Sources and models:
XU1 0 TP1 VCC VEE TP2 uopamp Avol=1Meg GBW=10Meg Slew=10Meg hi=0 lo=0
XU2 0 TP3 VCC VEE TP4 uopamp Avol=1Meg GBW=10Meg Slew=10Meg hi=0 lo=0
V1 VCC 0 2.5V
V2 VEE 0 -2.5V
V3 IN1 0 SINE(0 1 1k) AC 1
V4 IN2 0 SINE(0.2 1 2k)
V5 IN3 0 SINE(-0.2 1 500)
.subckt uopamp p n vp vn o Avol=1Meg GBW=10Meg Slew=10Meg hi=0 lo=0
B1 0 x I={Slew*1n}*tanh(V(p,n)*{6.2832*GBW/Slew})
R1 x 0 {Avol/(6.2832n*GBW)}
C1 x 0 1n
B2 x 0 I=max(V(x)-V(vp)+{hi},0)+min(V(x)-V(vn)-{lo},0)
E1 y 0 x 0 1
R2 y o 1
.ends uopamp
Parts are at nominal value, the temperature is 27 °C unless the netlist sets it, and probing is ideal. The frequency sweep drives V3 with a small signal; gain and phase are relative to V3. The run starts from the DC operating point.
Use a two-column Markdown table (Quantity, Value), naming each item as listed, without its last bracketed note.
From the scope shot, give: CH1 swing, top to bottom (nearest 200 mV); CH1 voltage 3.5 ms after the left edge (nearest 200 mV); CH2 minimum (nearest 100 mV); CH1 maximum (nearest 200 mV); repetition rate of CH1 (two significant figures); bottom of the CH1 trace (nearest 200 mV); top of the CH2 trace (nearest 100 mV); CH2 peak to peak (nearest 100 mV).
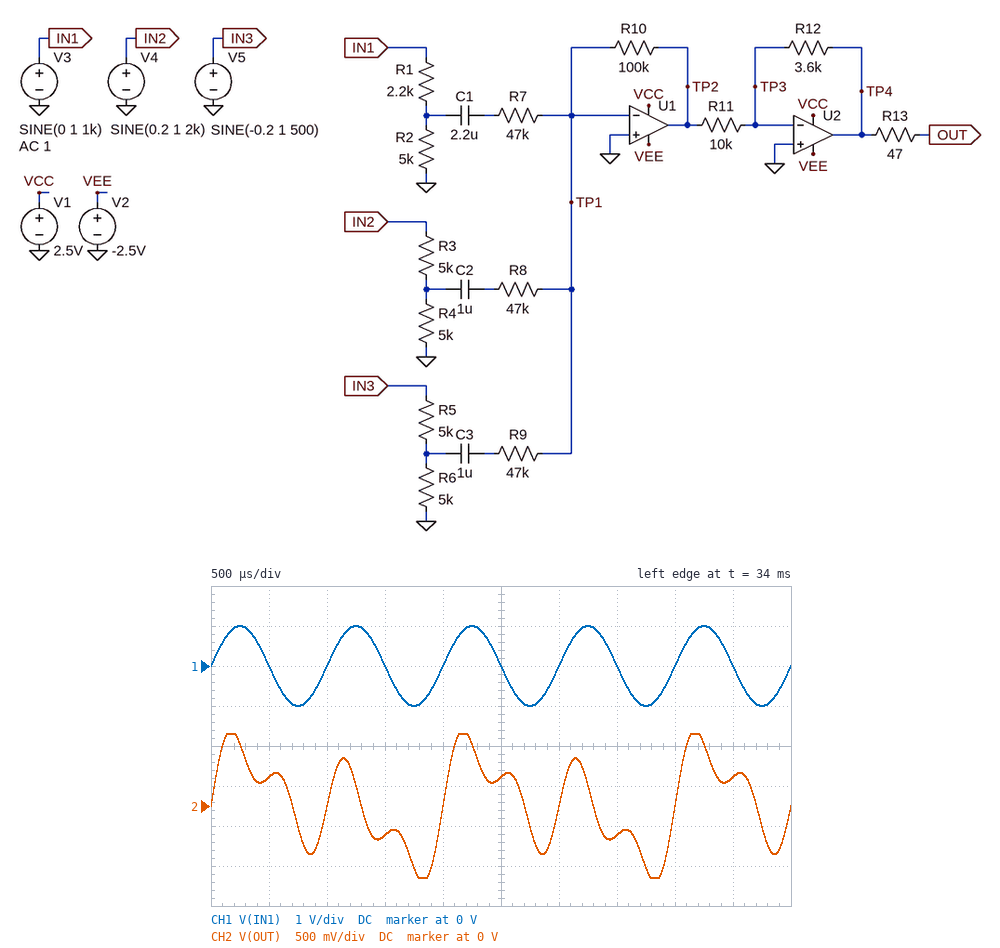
| Quantity | Value |
|---|---|
| CH1 swing, top to bottom | 2.0 V |
| CH1 voltage 3.5 ms after the left edge | 0 V |
| CH2 minimum | -900 mV |
| CH1 maximum | 1.0 V |
| repetition rate of CH1 | 1.0 kHz |
| bottom of the CH1 trace | -1.0 V |
| top of the CH2 trace | 900 mV |
| CH2 peak to peak | 1.8 V |
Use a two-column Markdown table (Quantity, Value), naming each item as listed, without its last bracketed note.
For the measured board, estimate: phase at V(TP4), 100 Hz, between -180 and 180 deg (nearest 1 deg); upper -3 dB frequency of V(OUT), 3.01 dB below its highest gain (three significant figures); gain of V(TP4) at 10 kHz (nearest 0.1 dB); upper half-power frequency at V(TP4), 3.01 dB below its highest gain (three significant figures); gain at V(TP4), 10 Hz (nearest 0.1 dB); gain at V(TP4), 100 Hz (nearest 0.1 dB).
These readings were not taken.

| Quantity | Value |
|---|---|
| phase at V(TP4), 100 Hz, between -180 and 180 deg | 1 deg |
| upper -3 dB frequency of V(OUT), 3.01 dB below its highest gain | 1.36 MHz |
| gain of V(TP4) at 10 kHz | -5.8 dB |
| upper half-power frequency at V(TP4), 3.01 dB below its highest gain | 1.36 MHz |
| gain at V(TP4), 10 Hz | -5.9 dB |
| gain at V(TP4), 100 Hz | -5.8 dB |
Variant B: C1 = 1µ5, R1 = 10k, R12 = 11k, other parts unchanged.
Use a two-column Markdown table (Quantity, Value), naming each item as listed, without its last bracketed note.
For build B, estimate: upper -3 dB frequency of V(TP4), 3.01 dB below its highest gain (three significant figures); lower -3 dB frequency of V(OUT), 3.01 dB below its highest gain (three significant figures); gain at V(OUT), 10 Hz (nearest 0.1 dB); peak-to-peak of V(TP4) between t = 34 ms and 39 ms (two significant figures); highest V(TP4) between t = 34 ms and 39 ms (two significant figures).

| Quantity | Value |
|---|---|
| upper -3 dB frequency of V(TP4), 3.01 dB below its highest gain | 1.32 MHz |
| lower -3 dB frequency of V(OUT), 3.01 dB below its highest gain | 2.11 Hz |
| gain at V(OUT), 10 Hz | -2.9 dB |
| peak-to-peak of V(TP4) between t = 34 ms and 39 ms | 4.3 V |
| highest V(TP4) between t = 34 ms and 39 ms | 2.2 V |
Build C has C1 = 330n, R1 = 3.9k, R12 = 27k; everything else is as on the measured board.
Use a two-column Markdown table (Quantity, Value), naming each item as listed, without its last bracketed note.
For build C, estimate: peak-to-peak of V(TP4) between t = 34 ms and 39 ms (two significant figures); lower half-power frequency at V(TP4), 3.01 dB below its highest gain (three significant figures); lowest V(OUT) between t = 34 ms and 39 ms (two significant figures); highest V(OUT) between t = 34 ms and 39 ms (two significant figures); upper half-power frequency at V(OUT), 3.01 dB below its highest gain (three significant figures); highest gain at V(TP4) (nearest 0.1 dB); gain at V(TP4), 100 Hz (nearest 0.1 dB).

| Quantity | Value |
|---|---|
| peak-to-peak of V(TP4) between t = 34 ms and 39 ms | 5.0 V |
| lower half-power frequency at V(TP4), 3.01 dB below its highest gain | 9.80 Hz |
| lowest V(OUT) between t = 34 ms and 39 ms | -2.5 V |
| highest V(OUT) between t = 34 ms and 39 ms | 2.5 V |
| upper half-power frequency at V(OUT), 3.01 dB below its highest gain | 1.17 MHz |
| highest gain at V(TP4) | 9.8 dB |
| gain at V(TP4), 100 Hz | 9.7 dB |
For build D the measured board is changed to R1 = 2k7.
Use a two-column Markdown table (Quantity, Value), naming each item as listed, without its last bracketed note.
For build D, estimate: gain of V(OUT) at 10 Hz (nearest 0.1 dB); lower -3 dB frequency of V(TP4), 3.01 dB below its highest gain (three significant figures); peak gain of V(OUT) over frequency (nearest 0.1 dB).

| Quantity | Value |
|---|---|
| gain of V(OUT) at 10 Hz | -6.5 dB |
| lower -3 dB frequency of V(TP4), 3.01 dB below its highest gain | 1.48 Hz |
| peak gain of V(OUT) over frequency | -6.4 dB |
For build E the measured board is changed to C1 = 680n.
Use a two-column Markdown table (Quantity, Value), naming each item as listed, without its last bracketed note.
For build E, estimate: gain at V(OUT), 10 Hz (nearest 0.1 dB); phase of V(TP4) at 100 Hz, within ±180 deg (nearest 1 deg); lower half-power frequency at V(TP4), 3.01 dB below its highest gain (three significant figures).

| Quantity | Value |
|---|---|
| gain at V(OUT), 10 Hz | -6.7 dB |
| phase of V(TP4) at 100 Hz, within ±180 deg | 3 deg |
| lower half-power frequency at V(TP4), 3.01 dB below its highest gain | 4.82 Hz |
